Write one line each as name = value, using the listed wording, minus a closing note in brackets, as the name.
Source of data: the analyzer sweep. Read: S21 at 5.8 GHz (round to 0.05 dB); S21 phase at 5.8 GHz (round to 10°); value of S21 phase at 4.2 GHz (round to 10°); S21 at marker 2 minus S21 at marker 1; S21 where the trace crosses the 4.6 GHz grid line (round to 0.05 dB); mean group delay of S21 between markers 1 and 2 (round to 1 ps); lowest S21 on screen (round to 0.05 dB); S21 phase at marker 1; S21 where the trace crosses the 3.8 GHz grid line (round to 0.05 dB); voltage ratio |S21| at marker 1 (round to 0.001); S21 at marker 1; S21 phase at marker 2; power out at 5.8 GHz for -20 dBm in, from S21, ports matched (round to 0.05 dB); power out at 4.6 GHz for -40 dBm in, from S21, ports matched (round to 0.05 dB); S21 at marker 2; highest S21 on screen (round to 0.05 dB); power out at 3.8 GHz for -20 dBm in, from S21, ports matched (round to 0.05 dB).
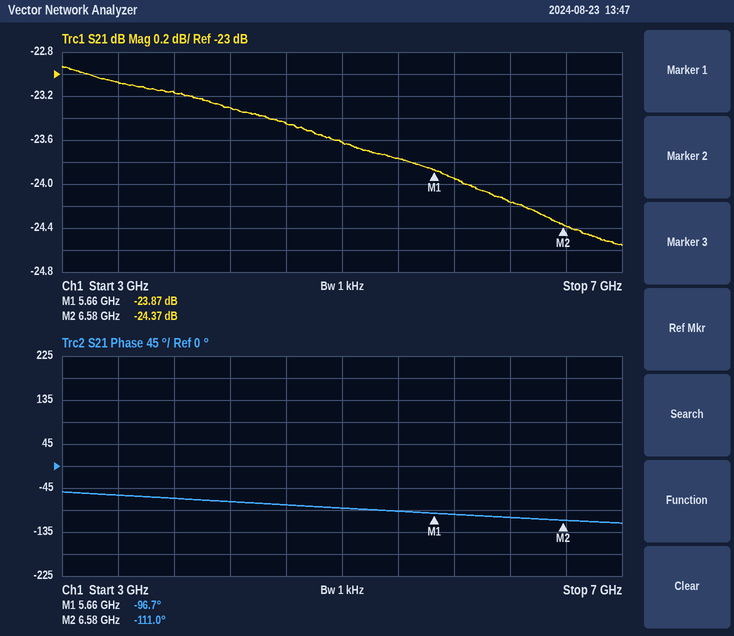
S21 at 5.8 GHz = -23.95 dB
S21 phase at 5.8 GHz = -100°
value of S21 phase at 4.2 GHz = -70°
S21 at marker 2 minus S21 at marker 1 = -0.50 dB
S21 where the trace crosses the 4.6 GHz grid line = -23.45 dB
mean group delay of S21 between markers 1 and 2 = 43 ps
lowest S21 on screen = -24.55 dB
S21 phase at marker 1 = -96.7°
S21 where the trace crosses the 3.8 GHz grid line = -23.15 dB
voltage ratio |S21| at marker 1 = 0.064
S21 at marker 1 = -23.87 dB
S21 phase at marker 2 = -111.0°
power out at 5.8 GHz for -20 dBm in, from S21, ports matched = -43.95 dBm
power out at 4.6 GHz for -40 dBm in, from S21, ports matched = -63.45 dBm
S21 at marker 2 = -24.37 dB
highest S21 on screen = -22.95 dB
power out at 3.8 GHz for -20 dBm in, from S21, ports matched = -43.15 dBm
